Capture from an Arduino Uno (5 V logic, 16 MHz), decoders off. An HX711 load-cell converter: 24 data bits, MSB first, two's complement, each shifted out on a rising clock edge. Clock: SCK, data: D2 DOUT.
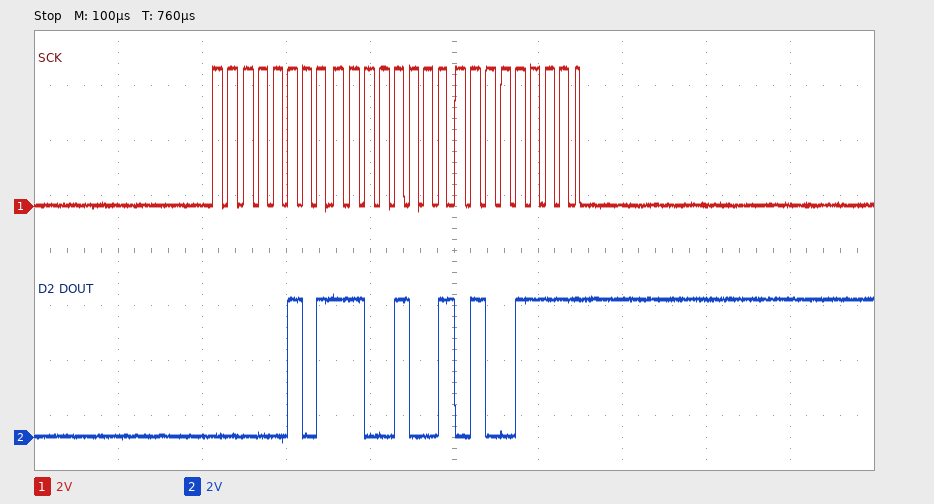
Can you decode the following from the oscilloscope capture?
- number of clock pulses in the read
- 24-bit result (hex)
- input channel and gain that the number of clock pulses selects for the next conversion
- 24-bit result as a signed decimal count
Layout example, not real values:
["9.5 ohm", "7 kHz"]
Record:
["25", "0x05C94F", "channel A, gain 128", "379215"]
